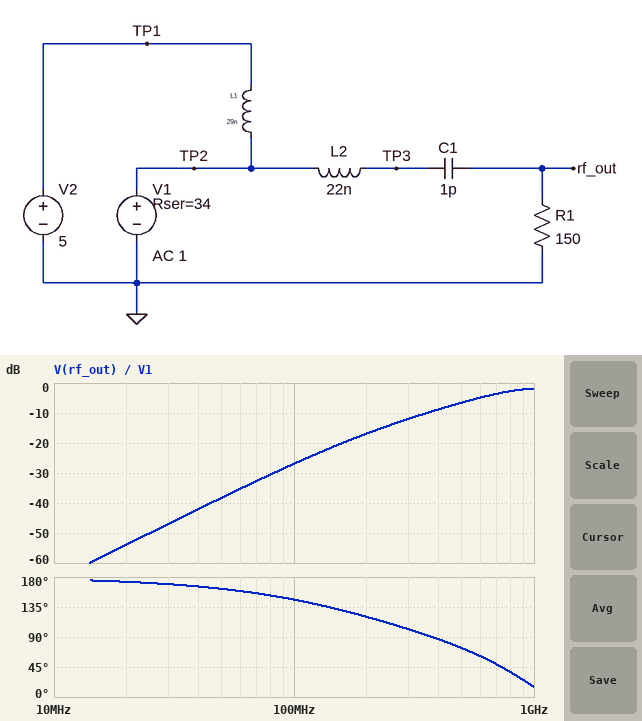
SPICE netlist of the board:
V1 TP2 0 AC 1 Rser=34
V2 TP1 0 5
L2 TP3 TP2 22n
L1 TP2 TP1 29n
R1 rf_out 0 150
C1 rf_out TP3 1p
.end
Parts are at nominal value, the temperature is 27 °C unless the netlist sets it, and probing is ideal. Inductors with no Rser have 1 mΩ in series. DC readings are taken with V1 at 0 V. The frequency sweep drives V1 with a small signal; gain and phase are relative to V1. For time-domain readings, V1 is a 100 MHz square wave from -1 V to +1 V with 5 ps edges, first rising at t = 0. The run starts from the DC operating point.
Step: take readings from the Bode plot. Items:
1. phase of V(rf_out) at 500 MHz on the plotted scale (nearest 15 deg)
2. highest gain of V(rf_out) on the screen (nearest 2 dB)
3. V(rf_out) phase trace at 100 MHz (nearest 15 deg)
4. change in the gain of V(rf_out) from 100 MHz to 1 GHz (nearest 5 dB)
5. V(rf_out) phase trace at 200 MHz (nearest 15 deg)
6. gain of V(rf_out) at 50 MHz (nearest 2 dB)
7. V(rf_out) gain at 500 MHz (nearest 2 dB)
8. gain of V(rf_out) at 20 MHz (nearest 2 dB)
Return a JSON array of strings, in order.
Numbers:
["75 deg", "-2 dB", "150 deg", "25 dB", "120 deg", "-38 dB", "-6 dB", "-54 dB"]
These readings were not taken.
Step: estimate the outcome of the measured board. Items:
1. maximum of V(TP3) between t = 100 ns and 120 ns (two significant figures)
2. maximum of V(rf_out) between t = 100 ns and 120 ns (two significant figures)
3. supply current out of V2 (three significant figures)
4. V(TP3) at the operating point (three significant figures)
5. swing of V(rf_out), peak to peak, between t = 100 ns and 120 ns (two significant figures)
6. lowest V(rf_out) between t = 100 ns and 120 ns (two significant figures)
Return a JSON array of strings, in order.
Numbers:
["6.9 V", "880 mV", "147 mA", "5.00 V", "1.8 V", "-880 mV"]
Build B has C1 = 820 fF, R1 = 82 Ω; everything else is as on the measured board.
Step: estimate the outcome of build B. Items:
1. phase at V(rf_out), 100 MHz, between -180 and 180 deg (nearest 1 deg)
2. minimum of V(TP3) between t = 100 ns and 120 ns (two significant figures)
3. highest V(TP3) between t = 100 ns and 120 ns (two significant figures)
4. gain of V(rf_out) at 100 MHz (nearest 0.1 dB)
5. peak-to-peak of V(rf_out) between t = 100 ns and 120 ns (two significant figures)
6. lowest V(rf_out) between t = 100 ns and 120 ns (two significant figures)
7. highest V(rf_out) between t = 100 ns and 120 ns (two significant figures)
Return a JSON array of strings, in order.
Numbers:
["149 deg", "2.8 V", "7.2 V", "-33.9 dB", "1.1 V", "-560 mV", "560 mV"]
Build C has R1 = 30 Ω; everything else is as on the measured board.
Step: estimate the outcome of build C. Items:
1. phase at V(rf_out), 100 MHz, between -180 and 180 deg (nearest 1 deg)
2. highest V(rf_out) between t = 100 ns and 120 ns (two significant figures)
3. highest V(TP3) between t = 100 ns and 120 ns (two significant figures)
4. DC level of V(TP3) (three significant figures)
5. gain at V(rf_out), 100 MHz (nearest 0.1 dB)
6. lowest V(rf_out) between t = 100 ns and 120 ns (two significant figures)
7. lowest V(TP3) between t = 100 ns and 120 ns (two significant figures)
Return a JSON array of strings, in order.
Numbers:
["150 deg", "260 mV", "7.4 V", "5.00 V", "-40.9 dB", "-260 mV", "2.6 V"]
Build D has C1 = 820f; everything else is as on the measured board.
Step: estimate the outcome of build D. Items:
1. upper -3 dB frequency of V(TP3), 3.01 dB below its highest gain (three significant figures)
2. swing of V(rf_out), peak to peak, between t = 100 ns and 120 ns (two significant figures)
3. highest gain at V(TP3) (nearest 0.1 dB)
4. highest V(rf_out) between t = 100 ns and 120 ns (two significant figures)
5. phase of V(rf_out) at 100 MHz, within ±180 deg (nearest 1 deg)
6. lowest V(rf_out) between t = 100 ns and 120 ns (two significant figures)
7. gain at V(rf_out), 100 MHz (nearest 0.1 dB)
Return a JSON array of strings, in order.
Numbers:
["1.61 GHz", "1.7 V", "2.1 dB", "850 mV", "147 deg", "-850 mV", "-28.7 dB"]
